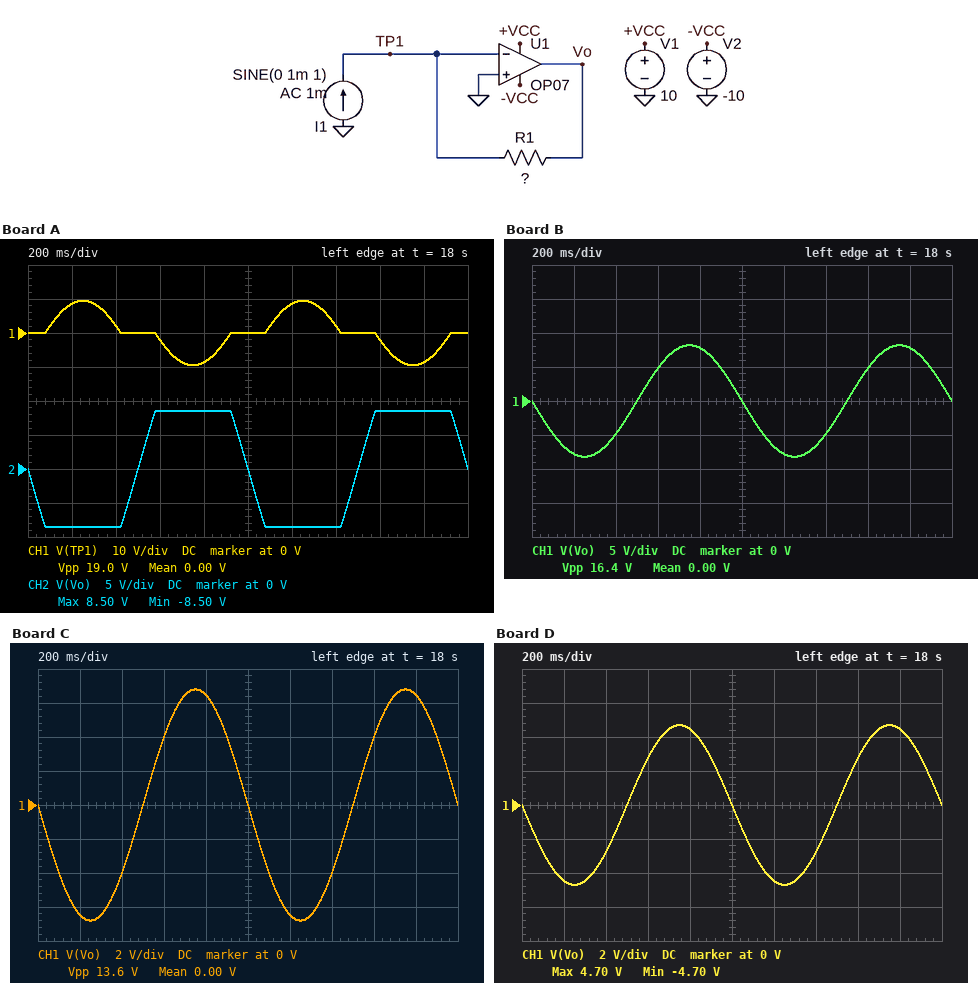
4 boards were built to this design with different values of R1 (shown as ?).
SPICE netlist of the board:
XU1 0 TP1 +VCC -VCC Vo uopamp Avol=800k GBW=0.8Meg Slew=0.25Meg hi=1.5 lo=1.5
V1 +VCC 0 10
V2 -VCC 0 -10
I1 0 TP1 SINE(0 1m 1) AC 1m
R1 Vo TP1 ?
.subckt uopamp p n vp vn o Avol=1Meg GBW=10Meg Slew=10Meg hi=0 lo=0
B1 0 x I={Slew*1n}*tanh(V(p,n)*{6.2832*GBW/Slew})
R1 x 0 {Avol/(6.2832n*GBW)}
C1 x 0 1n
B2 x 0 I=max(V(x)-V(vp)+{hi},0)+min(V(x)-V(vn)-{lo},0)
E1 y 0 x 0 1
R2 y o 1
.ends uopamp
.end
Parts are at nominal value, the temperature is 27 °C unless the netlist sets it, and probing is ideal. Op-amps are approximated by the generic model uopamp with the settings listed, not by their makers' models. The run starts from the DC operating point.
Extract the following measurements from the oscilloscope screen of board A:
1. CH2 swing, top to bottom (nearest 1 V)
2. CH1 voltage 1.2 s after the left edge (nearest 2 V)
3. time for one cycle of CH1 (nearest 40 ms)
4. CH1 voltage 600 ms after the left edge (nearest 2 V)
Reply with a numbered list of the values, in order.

1. 17 V
2. 8 V
3. 1.00 s
4. -2 V
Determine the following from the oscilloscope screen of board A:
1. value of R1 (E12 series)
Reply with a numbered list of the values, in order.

1. 18 kΩ
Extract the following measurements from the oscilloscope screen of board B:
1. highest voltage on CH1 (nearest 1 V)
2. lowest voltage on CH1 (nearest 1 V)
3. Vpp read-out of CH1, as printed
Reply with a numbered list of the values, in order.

1. 8 V
2. -8 V
3. 16.4 V
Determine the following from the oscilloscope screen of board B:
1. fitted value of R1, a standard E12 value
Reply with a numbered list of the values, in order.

1. 8.2 kΩ
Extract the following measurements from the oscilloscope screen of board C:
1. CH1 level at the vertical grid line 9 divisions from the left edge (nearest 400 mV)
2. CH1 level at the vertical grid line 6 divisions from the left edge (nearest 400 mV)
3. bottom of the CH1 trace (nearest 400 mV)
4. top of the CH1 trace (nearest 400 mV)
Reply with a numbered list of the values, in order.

1. 6.4 V
2. -6.4 V
3. -6.8 V
4. 6.8 V
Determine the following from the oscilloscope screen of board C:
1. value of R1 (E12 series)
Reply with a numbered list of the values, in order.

1. 6.8 kΩ
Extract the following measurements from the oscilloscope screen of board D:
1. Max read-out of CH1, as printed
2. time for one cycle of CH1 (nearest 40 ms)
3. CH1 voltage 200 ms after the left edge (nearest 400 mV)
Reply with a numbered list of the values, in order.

1. 4.70 V
2. 1.00 s
3. -4.4 V
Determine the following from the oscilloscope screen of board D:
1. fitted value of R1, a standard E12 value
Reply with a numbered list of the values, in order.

1. 4.7 kΩ
